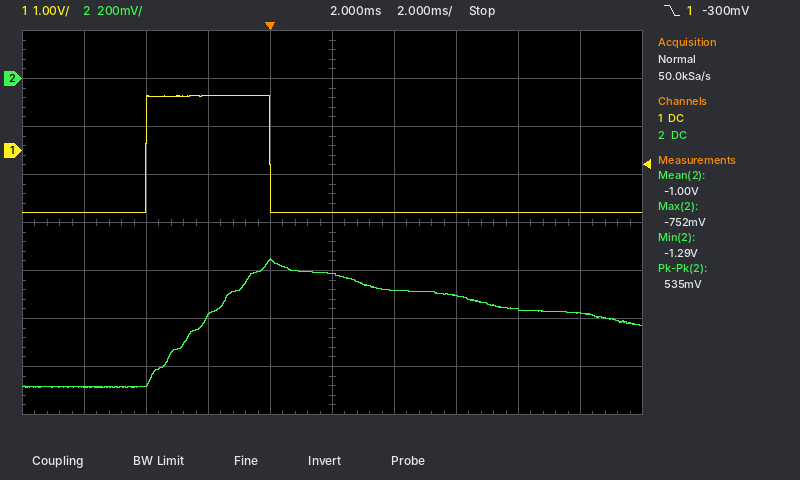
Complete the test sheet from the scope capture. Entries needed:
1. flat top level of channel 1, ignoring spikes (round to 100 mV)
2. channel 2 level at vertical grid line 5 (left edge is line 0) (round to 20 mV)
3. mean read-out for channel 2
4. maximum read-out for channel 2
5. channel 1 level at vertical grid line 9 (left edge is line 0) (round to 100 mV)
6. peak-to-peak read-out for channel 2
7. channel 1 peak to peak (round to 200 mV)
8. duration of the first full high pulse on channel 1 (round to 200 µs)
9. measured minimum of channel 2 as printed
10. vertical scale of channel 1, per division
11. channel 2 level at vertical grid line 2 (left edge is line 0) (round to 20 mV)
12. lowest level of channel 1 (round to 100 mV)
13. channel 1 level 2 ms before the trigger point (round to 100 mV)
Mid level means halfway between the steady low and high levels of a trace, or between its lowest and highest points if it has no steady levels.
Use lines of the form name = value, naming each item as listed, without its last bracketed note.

flat top level of channel 1, ignoring spikes = 1.1 V
channel 2 level at vertical grid line 5 (left edge is line 0) = -820 mV
mean read-out for channel 2 = -1.00 V
maximum read-out for channel 2 = -752 mV
channel 1 level at vertical grid line 9 (left edge is line 0) = -1.3 V
peak-to-peak read-out for channel 2 = 535 mV
channel 1 peak to peak = 2.4 V
duration of the first full high pulse on channel 1 = 4.0 ms
measured minimum of channel 2 as printed = -1.29 V
vertical scale of channel 1, per division = 1 V
channel 2 level at vertical grid line 2 (left edge is line 0) = -1.28 V
lowest level of channel 1 = -1.3 V
channel 1 level 2 ms before the trigger point = 1.1 V
